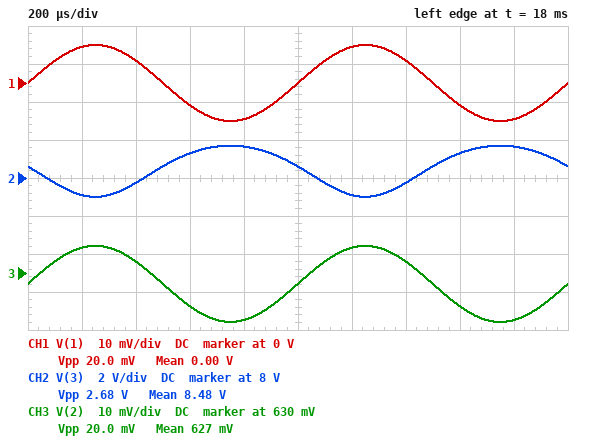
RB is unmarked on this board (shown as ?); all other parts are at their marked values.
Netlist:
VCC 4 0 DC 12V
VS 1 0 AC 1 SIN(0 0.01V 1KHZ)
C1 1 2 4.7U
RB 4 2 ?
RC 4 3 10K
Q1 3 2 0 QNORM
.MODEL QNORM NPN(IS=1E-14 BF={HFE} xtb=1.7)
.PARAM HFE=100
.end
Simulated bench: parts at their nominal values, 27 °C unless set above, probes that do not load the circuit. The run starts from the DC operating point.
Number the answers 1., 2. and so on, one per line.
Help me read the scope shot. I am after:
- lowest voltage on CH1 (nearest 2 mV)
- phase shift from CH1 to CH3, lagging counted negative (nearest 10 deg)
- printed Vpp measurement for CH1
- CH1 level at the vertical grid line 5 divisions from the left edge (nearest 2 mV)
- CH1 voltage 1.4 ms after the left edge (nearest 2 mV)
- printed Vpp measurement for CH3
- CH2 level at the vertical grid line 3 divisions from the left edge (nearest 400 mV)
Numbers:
1. -10 mV
2. 0 deg
3. 20.0 mV
4. 0 V
5. 6 mV
6. 20.0 mV
7. 9.2 V
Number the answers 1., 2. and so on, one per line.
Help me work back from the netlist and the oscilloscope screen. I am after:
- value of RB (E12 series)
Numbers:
1. 3.3 MΩ
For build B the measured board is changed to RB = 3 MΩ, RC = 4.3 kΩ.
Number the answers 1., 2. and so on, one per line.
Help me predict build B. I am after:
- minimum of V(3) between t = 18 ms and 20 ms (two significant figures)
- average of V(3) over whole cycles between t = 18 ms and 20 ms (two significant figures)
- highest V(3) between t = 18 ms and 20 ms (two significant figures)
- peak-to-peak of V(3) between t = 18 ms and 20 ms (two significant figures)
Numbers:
1. 9.6 V
2. 10 V
3. 11 V
4. 1.3 V
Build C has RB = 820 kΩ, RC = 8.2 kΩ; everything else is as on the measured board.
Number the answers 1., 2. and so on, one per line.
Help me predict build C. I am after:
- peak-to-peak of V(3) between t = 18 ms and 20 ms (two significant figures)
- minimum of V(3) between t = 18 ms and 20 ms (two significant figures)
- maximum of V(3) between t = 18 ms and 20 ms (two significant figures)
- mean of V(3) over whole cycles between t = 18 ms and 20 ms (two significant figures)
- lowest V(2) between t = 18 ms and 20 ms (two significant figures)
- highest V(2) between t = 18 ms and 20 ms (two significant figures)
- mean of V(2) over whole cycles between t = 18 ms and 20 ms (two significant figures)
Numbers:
1. 6.2 V
2. 100 mV
3. 6.3 V
4. 3.3 V
5. 650 mV
6. 670 mV
7. 660 mV
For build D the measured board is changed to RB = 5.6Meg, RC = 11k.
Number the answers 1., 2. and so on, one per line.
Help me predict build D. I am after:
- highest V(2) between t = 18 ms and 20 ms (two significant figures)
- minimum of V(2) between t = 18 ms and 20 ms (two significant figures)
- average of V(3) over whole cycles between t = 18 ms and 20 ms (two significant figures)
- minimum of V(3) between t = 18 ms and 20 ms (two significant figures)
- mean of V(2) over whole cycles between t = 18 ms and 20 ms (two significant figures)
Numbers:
1. 620 mV
2. 600 mV
3. 9.7 V
4. 8.7 V
5. 610 mV
